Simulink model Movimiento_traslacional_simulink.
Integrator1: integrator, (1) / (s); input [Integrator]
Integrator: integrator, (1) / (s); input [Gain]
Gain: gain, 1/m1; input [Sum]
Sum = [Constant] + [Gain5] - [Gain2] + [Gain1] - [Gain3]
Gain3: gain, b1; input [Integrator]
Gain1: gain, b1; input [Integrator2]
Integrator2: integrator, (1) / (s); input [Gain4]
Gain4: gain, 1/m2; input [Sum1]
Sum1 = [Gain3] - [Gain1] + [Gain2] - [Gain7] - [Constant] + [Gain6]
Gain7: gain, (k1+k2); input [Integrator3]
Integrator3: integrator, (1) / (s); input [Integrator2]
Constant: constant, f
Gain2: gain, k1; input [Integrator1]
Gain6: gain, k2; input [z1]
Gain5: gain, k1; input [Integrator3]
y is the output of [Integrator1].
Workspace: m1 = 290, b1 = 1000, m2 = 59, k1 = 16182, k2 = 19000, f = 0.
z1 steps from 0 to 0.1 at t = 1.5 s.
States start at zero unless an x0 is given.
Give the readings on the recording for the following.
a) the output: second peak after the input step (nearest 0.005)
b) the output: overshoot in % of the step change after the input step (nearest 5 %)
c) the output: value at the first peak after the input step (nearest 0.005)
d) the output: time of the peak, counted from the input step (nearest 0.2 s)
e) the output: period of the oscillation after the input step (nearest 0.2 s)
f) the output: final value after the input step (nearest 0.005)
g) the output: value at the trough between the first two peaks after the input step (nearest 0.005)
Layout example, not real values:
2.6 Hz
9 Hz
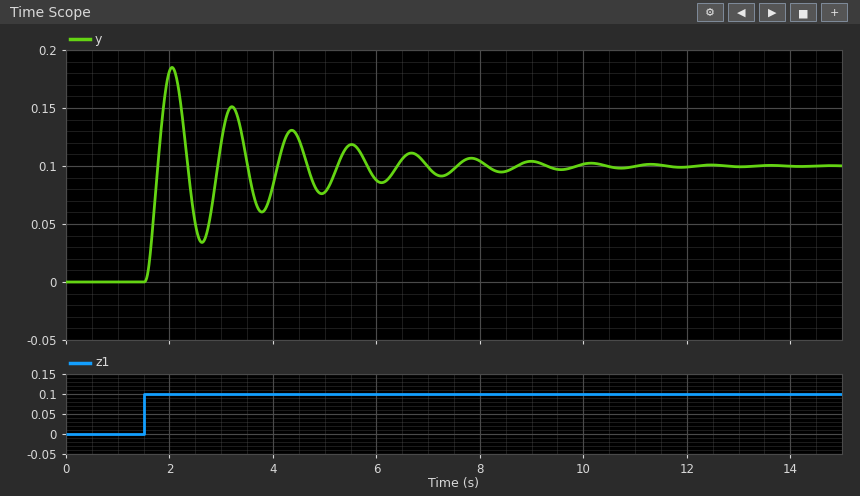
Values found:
0.150
85 %
0.185
0.6 s
1.2 s
0.100
0.035
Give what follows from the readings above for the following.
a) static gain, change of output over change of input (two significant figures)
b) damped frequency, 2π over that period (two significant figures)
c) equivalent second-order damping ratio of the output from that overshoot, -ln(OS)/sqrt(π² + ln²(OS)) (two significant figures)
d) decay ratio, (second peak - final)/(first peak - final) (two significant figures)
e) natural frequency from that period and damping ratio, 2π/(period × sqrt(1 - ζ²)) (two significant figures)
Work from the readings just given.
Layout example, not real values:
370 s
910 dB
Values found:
1.0
5.2 rad/s
0.052
0.59
5.2 rad/s
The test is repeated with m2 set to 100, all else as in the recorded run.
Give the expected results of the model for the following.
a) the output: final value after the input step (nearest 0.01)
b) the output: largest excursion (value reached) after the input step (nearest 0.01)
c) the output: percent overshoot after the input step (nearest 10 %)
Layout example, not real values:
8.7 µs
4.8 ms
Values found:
0.10
0.19
90 %
